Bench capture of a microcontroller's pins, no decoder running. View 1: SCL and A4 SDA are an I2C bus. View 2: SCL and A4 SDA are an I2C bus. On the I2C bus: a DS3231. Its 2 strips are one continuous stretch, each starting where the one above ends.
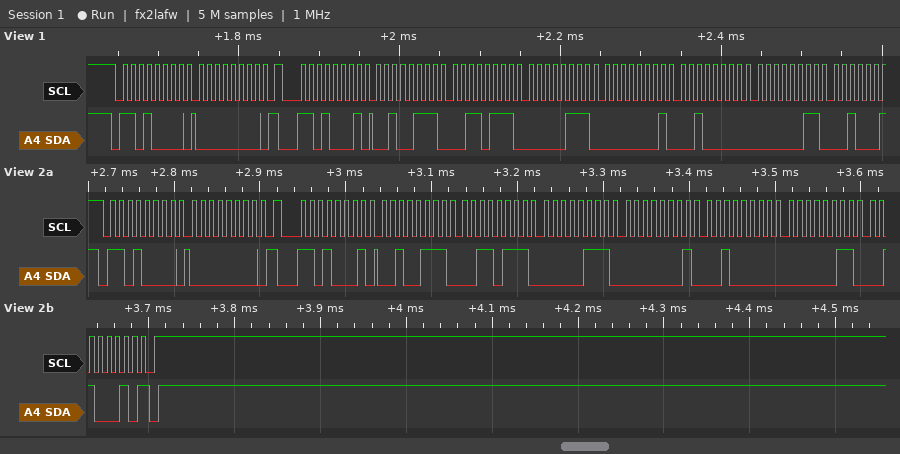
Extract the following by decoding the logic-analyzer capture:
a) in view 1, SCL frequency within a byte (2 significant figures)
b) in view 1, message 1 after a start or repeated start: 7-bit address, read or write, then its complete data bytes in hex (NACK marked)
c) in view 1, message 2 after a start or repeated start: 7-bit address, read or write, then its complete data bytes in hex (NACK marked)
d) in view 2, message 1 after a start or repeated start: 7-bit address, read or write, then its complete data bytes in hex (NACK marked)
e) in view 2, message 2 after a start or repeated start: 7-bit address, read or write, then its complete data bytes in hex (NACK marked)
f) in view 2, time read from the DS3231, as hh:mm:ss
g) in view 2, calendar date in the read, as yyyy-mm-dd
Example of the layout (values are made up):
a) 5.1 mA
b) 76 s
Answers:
a) 100 kHz
b) 0x68 write: 00
c) 0x68 read: 27 37 07 01 20 03
d) 0x68 write: 00
e) 0x68 read: 27 37 07 01 20 03 22 NACK
f) 07:37:27
g) 2022-03-20
